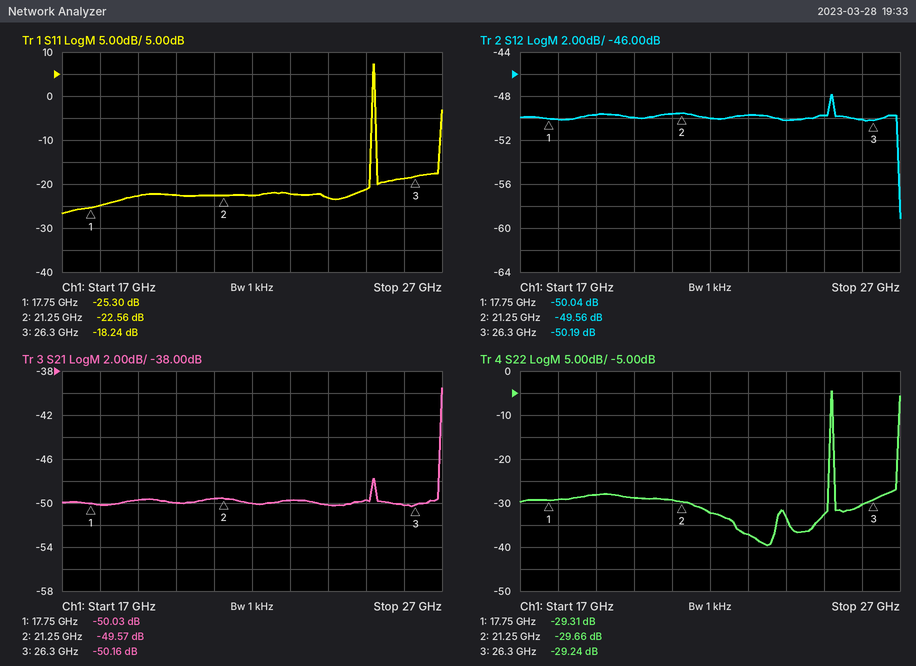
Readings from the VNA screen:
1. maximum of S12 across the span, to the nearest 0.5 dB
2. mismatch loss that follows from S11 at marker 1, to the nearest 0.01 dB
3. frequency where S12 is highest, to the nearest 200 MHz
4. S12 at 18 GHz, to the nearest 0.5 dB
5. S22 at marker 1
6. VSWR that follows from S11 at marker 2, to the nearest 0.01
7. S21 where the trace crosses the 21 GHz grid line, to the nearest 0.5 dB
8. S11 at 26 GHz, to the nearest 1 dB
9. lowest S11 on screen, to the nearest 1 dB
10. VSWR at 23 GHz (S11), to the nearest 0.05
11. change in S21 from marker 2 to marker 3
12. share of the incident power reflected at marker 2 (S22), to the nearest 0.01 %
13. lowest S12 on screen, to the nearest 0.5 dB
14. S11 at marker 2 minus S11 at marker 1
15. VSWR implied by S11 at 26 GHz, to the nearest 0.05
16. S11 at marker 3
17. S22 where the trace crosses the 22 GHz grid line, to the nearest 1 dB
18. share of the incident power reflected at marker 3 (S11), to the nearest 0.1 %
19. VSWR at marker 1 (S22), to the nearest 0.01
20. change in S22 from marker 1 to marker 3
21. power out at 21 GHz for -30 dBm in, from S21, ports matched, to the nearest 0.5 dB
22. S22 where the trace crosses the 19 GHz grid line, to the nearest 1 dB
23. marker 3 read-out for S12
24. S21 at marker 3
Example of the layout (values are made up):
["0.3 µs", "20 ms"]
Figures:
["-48.0 dB", "0.01 dB", "25.2 GHz", "-50.0 dB", "-29.31 dB", "1.16", "-49.5 dB", "-19 dB", "-27 dB", "1.15", "-0.59 dB", "0.11 %", "-59.0 dB", "2.74 dB", "1.25", "-18.24 dB", "-32 dB", "1.5 %", "1.07", "0.07 dB", "-79.5 dBm", "-28 dB", "-50.19 dB", "-50.16 dB"]
